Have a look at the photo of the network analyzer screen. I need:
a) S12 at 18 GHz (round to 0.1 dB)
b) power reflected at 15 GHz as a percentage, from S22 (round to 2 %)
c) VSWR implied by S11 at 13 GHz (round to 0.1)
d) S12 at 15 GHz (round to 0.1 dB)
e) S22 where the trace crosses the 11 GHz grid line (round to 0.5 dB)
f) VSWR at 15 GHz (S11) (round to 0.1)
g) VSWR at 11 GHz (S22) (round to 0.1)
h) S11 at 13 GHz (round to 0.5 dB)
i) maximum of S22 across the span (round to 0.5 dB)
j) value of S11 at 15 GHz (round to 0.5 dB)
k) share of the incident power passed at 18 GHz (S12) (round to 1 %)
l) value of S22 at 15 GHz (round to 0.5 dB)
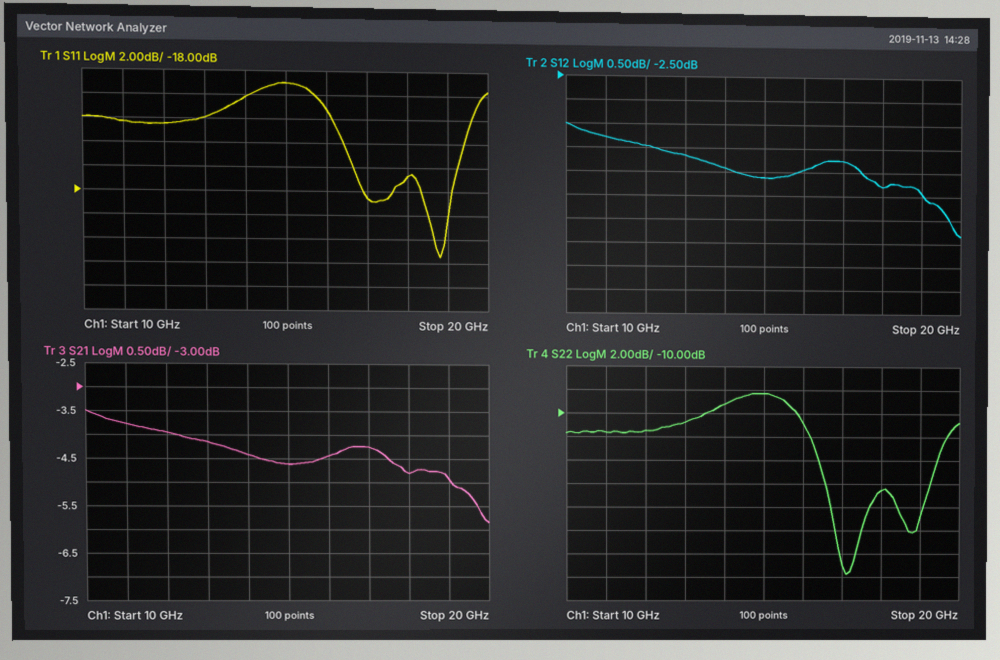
-4.8 dB
14 %
1.7
-4.6 dB
-11.5 dB
2.1
1.7
-12.0 dB
-8.5 dB
-9.0 dB
33 %
-8.5 dB
